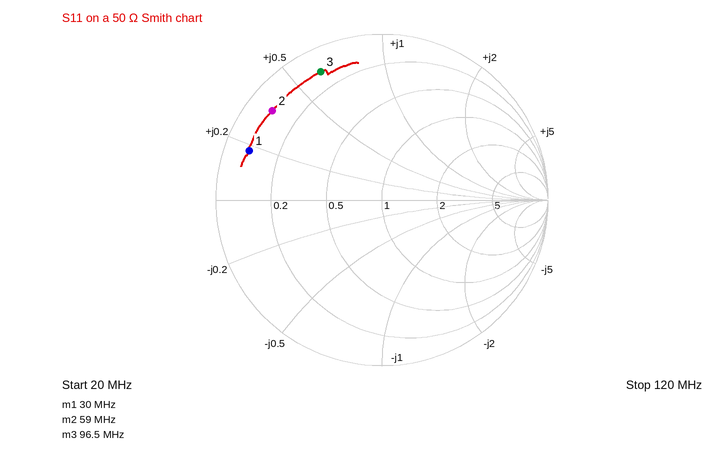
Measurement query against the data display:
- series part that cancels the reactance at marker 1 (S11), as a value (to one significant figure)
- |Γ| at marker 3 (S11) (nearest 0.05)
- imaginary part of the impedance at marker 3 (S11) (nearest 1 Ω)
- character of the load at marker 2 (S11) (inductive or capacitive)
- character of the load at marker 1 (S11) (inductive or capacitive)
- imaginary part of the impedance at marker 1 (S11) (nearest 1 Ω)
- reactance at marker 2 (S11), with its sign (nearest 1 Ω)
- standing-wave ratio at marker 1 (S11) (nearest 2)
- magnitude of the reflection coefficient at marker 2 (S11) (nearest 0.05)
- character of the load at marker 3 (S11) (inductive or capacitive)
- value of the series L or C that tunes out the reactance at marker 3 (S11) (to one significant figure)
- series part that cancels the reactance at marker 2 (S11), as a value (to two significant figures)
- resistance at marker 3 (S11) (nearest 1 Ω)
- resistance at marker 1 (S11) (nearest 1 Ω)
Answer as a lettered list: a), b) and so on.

a) 600 pF
b) 0.85
c) +31 Ω
d) inductive
e) inductive
f) +9 Ω
g) +18 Ω
h) 12
i) 0.85
j) inductive
k) 50 pF
l) 150 pF
m) 5 Ω
n) 4 Ω
